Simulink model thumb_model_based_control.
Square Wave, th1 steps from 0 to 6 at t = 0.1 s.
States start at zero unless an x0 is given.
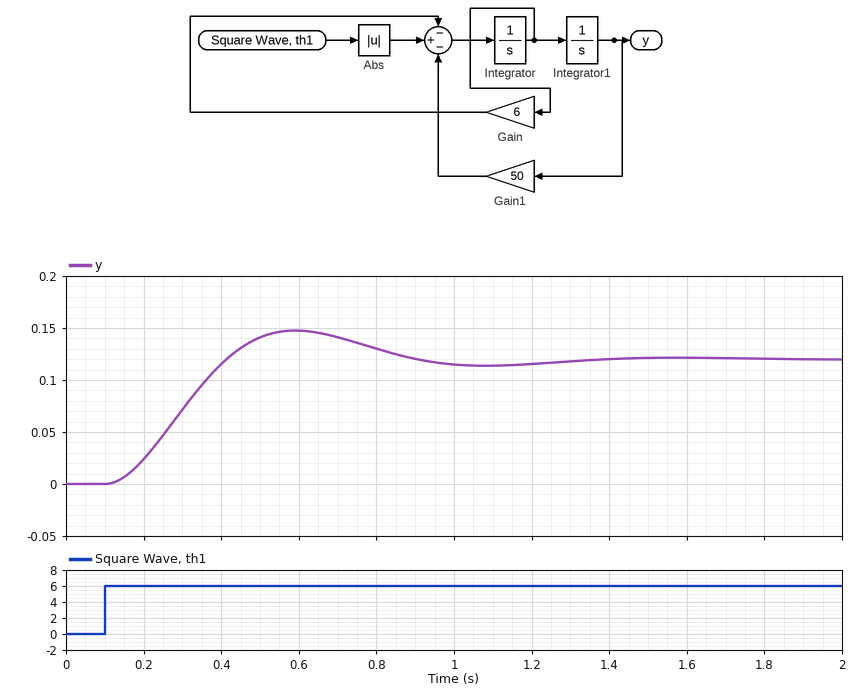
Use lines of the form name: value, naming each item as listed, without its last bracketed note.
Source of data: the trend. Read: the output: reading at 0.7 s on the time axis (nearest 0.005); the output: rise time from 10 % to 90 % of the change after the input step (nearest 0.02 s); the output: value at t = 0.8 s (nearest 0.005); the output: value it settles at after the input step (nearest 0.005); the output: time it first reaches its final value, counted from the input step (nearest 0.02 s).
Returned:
the output: reading at 0.7 s on the time axis: 0.140
the output: rise time from 10 % to 90 % of the change after the input step: 0.22 s
the output: value at t = 0.8 s: 0.130
the output: value it settles at after the input step: 0.120
the output: time it first reaches its final value, counted from the input step: 0.32 s
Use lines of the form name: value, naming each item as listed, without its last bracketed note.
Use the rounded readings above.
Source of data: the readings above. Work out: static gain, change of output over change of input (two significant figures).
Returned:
static gain, change of output over change of input: 0.020
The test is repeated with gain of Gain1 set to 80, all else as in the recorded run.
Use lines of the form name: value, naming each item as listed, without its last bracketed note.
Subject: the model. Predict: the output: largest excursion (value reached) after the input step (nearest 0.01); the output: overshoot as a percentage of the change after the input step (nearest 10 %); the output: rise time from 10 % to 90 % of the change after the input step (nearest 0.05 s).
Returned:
the output: largest excursion (value reached) after the input step: 0.10
the output: overshoot as a percentage of the change after the input step: 30 %
the output: rise time from 10 % to 90 % of the change after the input step: 0.15 s
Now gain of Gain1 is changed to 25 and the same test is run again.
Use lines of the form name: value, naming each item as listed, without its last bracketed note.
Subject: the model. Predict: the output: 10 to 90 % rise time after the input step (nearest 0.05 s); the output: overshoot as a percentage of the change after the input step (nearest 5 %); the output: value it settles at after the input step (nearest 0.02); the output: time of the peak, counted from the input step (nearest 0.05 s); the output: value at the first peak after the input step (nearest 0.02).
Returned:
the output: 10 to 90 % rise time after the input step: 0.35 s
the output: overshoot as a percentage of the change after the input step: 10 %
the output: value it settles at after the input step: 0.24
the output: time of the peak, counted from the input step: 0.80 s
the output: value at the first peak after the input step: 0.26
